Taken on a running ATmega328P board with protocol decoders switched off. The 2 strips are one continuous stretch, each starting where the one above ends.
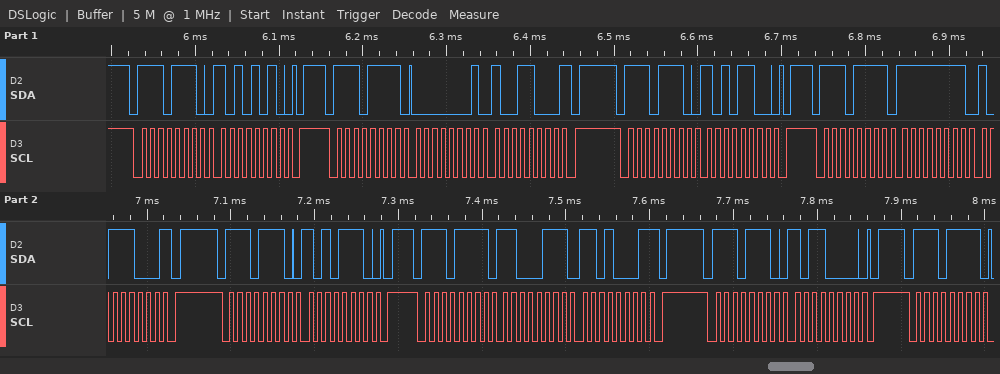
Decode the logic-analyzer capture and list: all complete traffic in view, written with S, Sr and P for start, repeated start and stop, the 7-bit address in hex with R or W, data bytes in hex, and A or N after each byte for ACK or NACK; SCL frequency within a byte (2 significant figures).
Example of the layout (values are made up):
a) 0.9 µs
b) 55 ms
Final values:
a) S 77W A AA A P S 77R A 01 A 98 N P S 77W A AC A P S 77R A FF A B8 N P S 77W A AE A P S 77R A C7 A D1 N P S 77W A B0 A P S 77R A
b) 100 kHz
